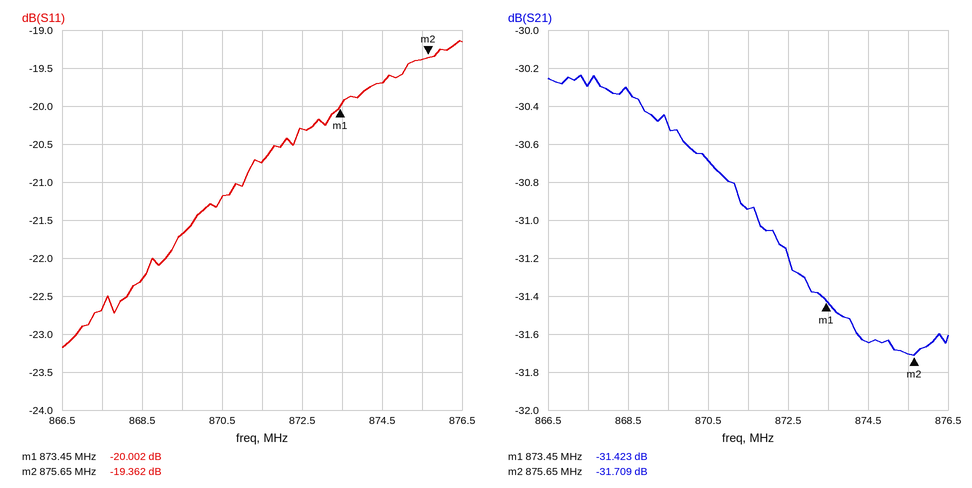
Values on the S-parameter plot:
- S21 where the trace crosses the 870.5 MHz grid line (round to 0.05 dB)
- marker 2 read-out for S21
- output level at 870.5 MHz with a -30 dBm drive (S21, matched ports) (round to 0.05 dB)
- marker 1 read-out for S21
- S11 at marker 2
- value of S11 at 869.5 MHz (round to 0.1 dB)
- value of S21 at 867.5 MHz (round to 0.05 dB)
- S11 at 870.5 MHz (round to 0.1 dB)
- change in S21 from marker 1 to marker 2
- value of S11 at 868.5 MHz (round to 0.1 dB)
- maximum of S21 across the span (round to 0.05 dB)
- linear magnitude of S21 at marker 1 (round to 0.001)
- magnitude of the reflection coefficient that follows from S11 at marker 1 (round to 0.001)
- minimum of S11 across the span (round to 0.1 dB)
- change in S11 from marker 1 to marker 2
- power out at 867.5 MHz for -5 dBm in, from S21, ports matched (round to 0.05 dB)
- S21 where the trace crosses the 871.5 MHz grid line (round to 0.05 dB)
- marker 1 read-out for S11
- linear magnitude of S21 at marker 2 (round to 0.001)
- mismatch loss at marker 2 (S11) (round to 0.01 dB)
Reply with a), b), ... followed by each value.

a) -30.70 dB
b) -31.709 dB
c) -60.70 dBm
d) -31.423 dB
e) -19.362 dB
f) -21.7 dB
g) -30.30 dB
h) -21.2 dB
i) -0.286 dB
j) -22.3 dB
k) -30.25 dB
l) 0.027
m) 0.100
n) -23.2 dB
o) 0.640 dB
p) -35.30 dBm
q) -30.95 dB
r) -20.002 dB
s) 0.026
t) 0.05 dB
